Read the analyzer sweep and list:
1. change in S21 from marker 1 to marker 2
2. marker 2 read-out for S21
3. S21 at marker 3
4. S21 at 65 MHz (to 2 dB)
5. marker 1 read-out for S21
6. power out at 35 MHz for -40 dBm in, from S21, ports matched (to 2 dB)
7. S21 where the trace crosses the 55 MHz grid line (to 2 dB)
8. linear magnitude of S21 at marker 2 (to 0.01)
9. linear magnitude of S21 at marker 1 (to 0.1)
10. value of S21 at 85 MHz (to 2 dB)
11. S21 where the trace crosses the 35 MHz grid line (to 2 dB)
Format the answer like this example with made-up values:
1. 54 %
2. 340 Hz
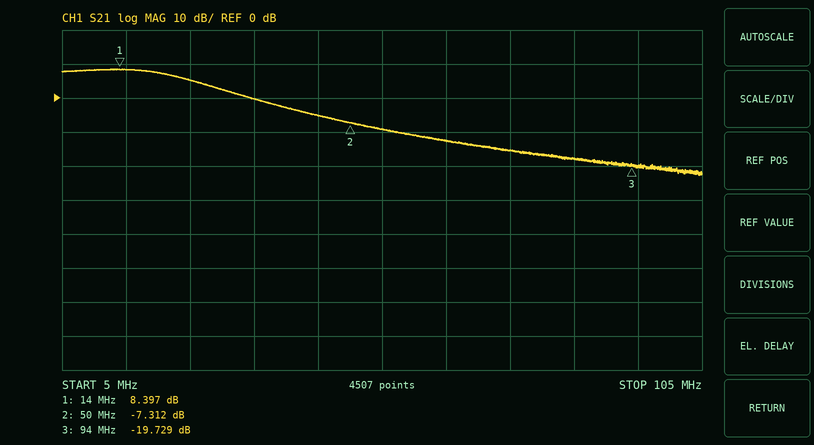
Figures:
1. -15.709 dB
2. -7.312 dB
3. -19.729 dB
4. -12 dB
5. 8.397 dB
6. -40 dBm
7. -10 dB
8. 0.43
9. 2.6
10. -18 dB
11. 0 dB
